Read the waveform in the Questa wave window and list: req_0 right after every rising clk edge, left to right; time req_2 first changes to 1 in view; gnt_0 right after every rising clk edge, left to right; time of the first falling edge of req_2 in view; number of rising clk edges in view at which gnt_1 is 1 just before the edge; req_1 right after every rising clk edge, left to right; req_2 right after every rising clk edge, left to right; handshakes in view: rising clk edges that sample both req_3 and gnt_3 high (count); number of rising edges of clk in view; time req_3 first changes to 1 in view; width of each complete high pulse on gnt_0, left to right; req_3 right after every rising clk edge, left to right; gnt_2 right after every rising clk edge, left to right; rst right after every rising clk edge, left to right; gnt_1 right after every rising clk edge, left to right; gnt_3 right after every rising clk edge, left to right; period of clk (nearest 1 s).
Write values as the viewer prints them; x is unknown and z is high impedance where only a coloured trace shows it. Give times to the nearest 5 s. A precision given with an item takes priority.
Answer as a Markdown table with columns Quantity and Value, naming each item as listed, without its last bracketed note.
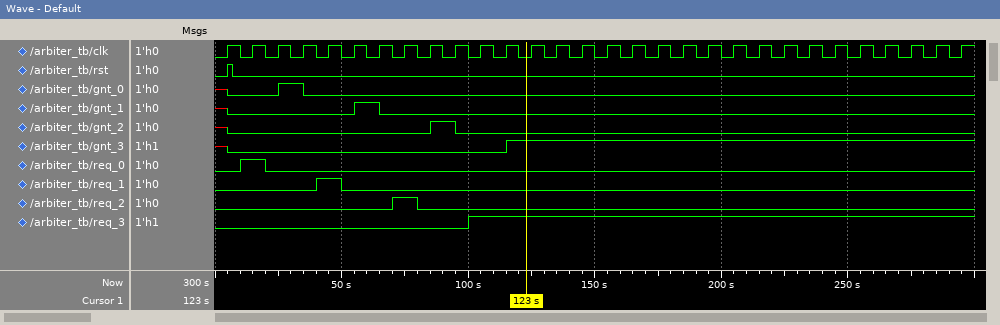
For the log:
| Quantity | Value |
|---|---|
| req_0 right after every rising clk edge, left to right | 0 1 0 0 0 0 0 0 0 0 0 0 0 0 0 0 0 0 0 0 0 0 0 0 0 0 0 0 0 0 |
| time req_2 first changes to 1 in view | 70 s |
| gnt_0 right after every rising clk edge, left to right | 0 0 1 0 0 0 0 0 0 0 0 0 0 0 0 0 0 0 0 0 0 0 0 0 0 0 0 0 0 0 |
| time of the first falling edge of req_2 in view | 80 s |
| number of rising clk edges in view at which gnt_1 is 1 just before the edge | 1 |
| req_1 right after every rising clk edge, left to right | 0 0 0 0 1 0 0 0 0 0 0 0 0 0 0 0 0 0 0 0 0 0 0 0 0 0 0 0 0 0 |
| req_2 right after every rising clk edge, left to right | 0 0 0 0 0 0 0 1 0 0 0 0 0 0 0 0 0 0 0 0 0 0 0 0 0 0 0 0 0 0 |
| handshakes in view: rising clk edges that sample both req_3 and gnt_3 high | 18 |
| number of rising edges of clk in view | 30 |
| time req_3 first changes to 1 in view | 100 s |
| width of each complete high pulse on gnt_0, left to right | 10 s |
| req_3 right after every rising clk edge, left to right | 0 0 0 0 0 0 0 0 0 0 1 1 1 1 1 1 1 1 1 1 1 1 1 1 1 1 1 1 1 1 |
| gnt_2 right after every rising clk edge, left to right | 0 0 0 0 0 0 0 0 1 0 0 0 0 0 0 0 0 0 0 0 0 0 0 0 0 0 0 0 0 0 |
| rst right after every rising clk edge, left to right | 1 0 0 0 0 0 0 0 0 0 0 0 0 0 0 0 0 0 0 0 0 0 0 0 0 0 0 0 0 0 |
| gnt_1 right after every rising clk edge, left to right | 0 0 0 0 0 1 0 0 0 0 0 0 0 0 0 0 0 0 0 0 0 0 0 0 0 0 0 0 0 0 |
| gnt_3 right after every rising clk edge, left to right | 0 0 0 0 0 0 0 0 0 0 0 1 1 1 1 1 1 1 1 1 1 1 1 1 1 1 1 1 1 1 |
| period of clk | 10 s |
